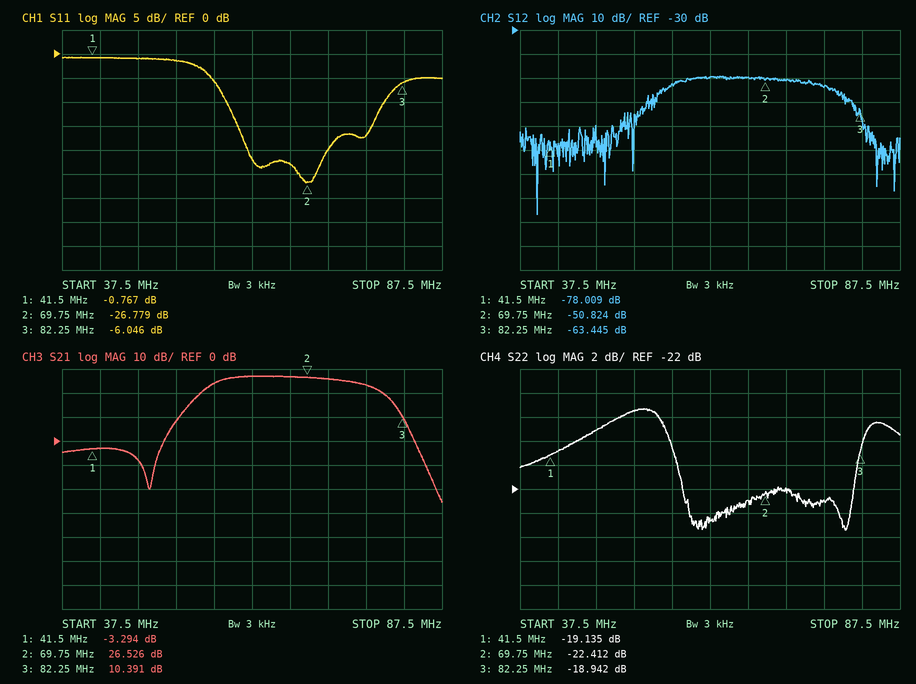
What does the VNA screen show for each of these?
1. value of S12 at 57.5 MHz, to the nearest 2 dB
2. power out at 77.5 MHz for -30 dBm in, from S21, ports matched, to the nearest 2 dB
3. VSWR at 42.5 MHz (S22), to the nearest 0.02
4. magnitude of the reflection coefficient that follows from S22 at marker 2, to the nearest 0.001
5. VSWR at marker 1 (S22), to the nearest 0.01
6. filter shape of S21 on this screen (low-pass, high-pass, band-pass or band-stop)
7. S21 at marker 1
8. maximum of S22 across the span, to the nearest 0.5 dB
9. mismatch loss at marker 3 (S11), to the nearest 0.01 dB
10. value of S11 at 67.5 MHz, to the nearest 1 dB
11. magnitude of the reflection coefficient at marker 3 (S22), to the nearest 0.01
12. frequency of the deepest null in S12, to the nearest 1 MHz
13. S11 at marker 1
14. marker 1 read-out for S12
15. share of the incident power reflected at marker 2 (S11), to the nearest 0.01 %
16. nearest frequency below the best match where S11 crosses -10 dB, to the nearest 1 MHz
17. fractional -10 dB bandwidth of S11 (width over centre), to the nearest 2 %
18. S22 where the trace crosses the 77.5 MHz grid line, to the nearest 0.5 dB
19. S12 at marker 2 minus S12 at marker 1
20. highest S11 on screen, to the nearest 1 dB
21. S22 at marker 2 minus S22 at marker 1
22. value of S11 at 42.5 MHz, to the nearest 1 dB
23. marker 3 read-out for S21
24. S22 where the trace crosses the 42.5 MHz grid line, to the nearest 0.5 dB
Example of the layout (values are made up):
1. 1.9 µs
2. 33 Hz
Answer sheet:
1. -52 dB
2. -6 dBm
3. 1.26
4. 0.076
5. 1.25
6. band-pass
7. -3.294 dB
8. -15.5 dB
9. 1.24 dB
10. -23 dB
11. 0.11
12. 40 MHz
13. -0.767 dB
14. -78.009 dB
15. 0.21 %
16. 59 MHz
17. 30 %
18. -23.0 dB
19. 27.185 dB
20. -1 dB
21. -3.277 dB
22. -1 dB
23. 10.391 dB
24. -19.0 dB
